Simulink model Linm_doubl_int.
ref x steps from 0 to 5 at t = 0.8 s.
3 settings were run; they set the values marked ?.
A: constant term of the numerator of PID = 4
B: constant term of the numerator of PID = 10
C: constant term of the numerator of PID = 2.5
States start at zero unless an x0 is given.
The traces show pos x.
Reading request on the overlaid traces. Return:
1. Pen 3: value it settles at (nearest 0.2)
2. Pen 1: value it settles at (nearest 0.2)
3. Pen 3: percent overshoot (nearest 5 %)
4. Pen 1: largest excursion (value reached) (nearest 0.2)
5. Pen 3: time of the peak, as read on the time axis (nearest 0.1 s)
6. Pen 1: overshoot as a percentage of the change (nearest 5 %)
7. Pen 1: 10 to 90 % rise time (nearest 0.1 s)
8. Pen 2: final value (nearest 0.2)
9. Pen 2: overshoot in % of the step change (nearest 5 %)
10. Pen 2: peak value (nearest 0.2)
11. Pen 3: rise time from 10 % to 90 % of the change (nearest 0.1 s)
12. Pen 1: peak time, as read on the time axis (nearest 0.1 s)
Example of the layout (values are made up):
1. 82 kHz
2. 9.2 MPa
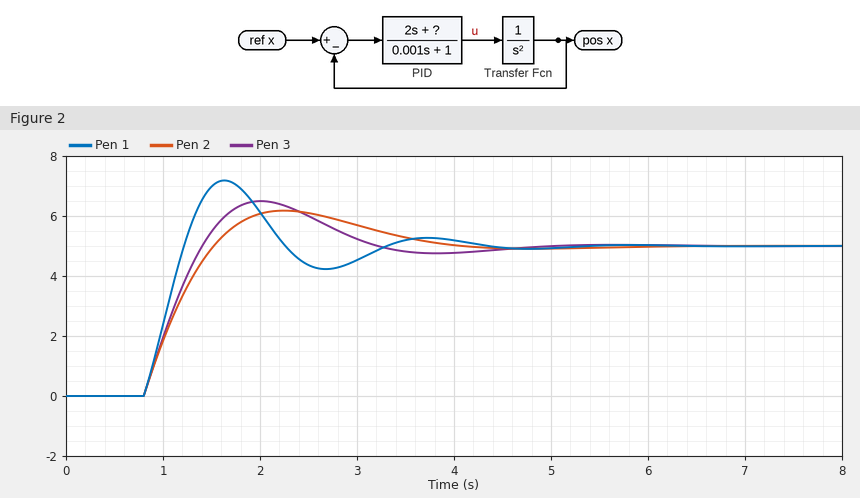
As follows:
1. 5.0
2. 5.0
3. 30 %
4. 7.2
5. 2.0 s
6. 45 %
7. 0.3 s
8. 5.0
9. 25 %
10. 6.2
11. 0.5 s
12. 1.6 s
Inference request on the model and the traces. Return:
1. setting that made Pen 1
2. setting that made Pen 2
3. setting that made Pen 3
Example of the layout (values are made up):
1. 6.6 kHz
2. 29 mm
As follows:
1. B
2. C
3. A
